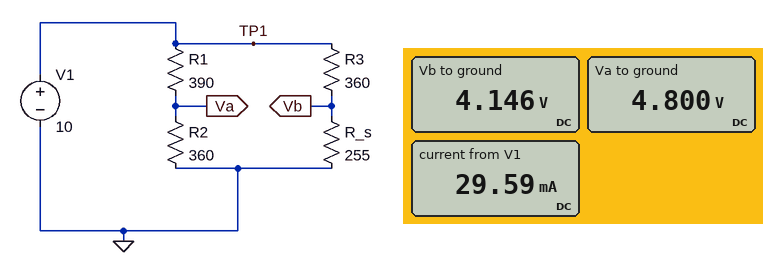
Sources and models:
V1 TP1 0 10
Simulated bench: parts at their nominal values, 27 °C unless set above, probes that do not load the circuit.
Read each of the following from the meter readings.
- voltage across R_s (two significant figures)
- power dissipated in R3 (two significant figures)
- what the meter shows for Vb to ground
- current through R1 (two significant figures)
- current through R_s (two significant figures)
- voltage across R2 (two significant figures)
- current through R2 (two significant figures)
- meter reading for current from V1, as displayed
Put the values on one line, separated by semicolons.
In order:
4.1 V; 95 mW; 4.146 V; 13 mA; 16 mA; 4.8 V; 13 mA; 29.59 mA
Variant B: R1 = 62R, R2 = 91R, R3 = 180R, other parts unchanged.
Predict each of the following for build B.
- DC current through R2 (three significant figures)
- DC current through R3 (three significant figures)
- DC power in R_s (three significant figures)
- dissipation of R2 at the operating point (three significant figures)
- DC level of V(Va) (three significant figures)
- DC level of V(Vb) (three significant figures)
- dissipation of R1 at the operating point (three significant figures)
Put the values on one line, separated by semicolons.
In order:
65.4 mA; 23.0 mA; 135 mW; 389 mW; 5.95 V; 5.86 V; 265 mW
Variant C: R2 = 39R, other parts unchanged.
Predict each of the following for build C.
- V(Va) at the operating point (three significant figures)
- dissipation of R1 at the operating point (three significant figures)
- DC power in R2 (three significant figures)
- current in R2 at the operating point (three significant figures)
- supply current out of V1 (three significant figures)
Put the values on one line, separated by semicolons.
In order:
909 mV; 212 mW; 21.2 mW; 23.3 mA; 39.6 mA
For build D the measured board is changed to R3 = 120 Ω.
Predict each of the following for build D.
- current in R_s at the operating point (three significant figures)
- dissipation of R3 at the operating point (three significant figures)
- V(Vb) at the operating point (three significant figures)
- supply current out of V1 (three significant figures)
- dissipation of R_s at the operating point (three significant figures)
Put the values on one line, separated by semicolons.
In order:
26.7 mA; 85.3 mW; 6.80 V; 40.0 mA; 181 mW
